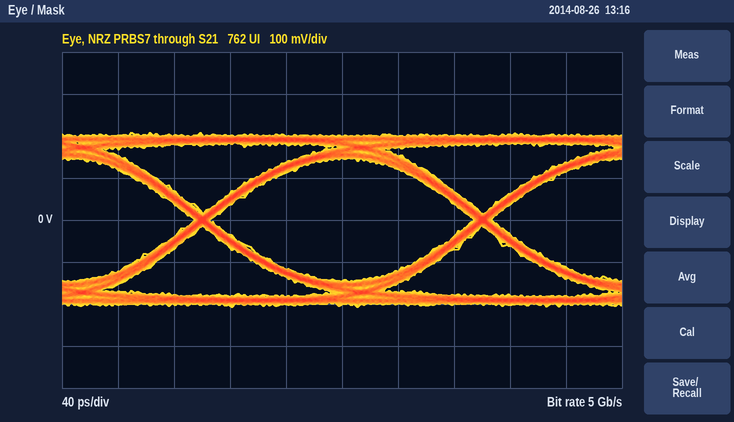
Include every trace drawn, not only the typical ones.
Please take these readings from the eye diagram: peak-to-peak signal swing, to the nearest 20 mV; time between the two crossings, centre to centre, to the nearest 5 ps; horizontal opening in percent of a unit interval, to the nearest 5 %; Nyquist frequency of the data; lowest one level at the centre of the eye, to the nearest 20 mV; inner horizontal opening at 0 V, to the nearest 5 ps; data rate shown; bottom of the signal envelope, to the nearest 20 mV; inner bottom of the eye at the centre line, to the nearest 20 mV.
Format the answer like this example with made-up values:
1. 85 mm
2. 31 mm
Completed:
1. 420 mV
2. 200 ps
3. 95 %
4. 2.5 GHz
5. 140 mV
6. 190 ps
7. 5 Gb/s
8. -200 mV
9. -140 mV
